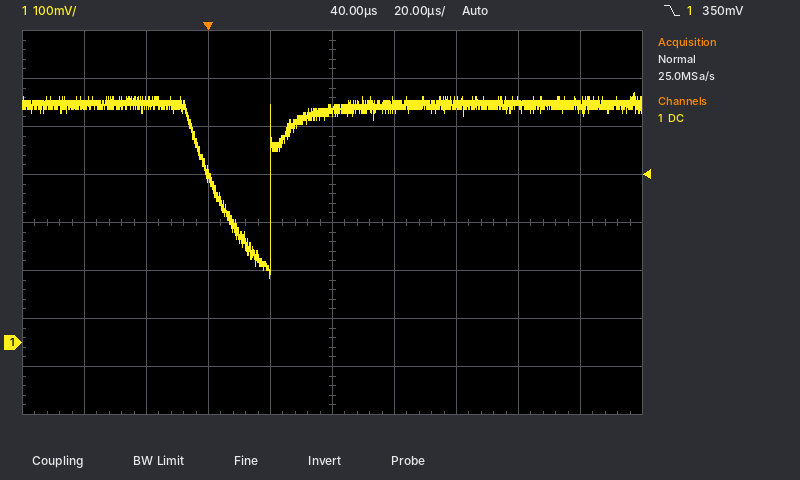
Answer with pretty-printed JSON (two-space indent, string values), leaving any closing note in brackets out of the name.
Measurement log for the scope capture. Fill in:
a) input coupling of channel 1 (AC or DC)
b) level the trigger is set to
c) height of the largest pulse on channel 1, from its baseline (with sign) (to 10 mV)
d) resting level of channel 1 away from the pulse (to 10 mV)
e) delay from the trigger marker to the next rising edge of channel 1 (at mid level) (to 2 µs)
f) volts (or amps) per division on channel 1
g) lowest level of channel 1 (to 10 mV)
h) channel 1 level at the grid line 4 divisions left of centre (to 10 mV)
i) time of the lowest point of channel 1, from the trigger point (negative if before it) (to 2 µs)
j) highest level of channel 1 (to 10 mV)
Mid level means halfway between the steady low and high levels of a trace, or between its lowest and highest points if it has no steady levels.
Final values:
{
  "input coupling of channel 1": "DC",
  "level the trigger is set to": "350 mV",
  "height of the largest pulse on channel 1, from its baseline (with sign)": "-360 mV",
  "resting level of channel 1 away from the pulse": "500 mV",
  "delay from the trigger marker to the next rising edge of channel 1 (at mid level)": "20 µs",
  "volts (or amps) per division on channel 1": "100 mV",
  "lowest level of channel 1": "140 mV",
  "channel 1 level at the grid line 4 divisions left of centre": "500 mV",
  "time of the lowest point of channel 1, from the trigger point (negative if before it)": "+20 µs",
  "highest level of channel 1": "520 mV"
}
